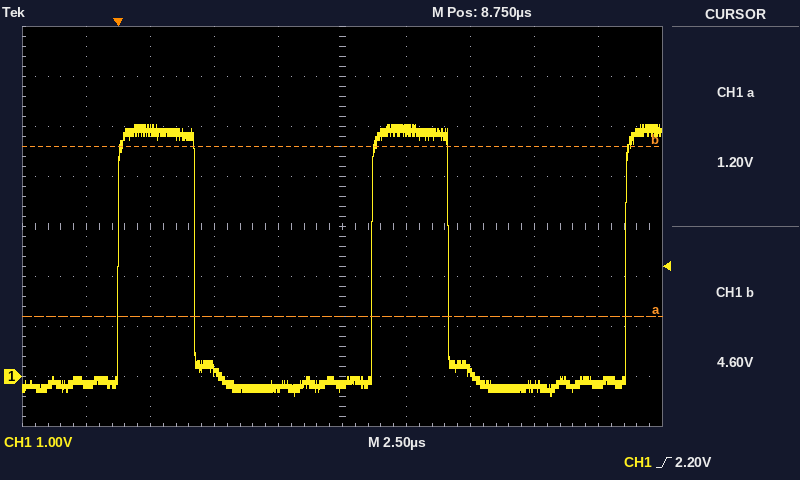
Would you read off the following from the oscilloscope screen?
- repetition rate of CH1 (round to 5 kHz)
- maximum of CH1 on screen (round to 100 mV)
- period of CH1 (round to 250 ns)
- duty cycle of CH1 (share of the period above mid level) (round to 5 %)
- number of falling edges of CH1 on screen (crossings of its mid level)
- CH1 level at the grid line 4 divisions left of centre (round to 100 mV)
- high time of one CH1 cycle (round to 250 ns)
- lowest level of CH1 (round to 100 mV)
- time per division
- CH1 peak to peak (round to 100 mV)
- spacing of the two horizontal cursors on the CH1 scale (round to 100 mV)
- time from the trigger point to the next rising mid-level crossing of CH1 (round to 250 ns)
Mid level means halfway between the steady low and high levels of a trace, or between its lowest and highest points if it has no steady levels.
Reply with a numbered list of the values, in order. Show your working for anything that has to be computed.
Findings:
1. 1 / 10.00 µs ≈ 100 kHz
2. 5.0 V
3. 10.00 µs
4. 3.00 µs / 10.00 µs ≈ 30 %
5. 2
6. -200 mV
7. 3.00 µs
8. -400 mV
9. 2.5 µs
10. 5.0 V − (-400 mV) = 5.4 V
11. 3.4 V
12. 10.00 µs
